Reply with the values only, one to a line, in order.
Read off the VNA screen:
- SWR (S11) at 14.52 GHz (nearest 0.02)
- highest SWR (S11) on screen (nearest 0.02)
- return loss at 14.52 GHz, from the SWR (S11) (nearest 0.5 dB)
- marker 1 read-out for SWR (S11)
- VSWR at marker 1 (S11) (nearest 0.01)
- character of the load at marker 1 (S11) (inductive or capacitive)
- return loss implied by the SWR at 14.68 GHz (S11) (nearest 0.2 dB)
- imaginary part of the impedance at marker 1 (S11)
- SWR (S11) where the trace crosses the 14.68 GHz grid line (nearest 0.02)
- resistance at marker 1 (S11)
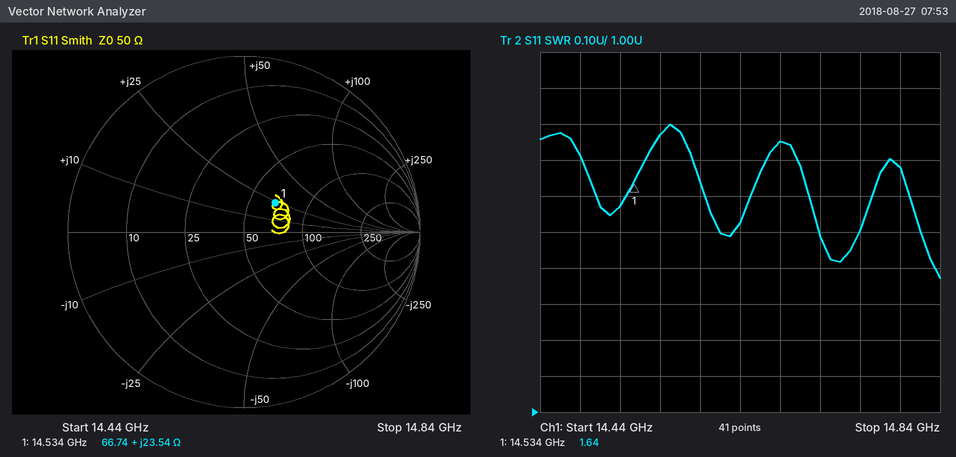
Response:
1.58
1.80
13.0 dB
1.64
1.64
inductive
11.2 dB
+23.54 Ω
1.76
66.74 Ω
